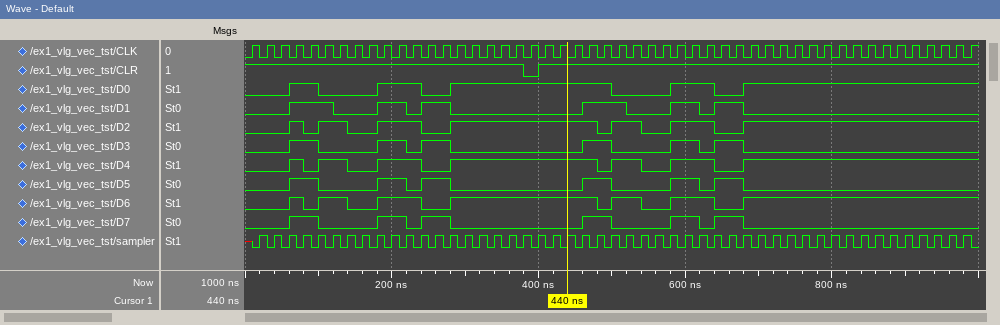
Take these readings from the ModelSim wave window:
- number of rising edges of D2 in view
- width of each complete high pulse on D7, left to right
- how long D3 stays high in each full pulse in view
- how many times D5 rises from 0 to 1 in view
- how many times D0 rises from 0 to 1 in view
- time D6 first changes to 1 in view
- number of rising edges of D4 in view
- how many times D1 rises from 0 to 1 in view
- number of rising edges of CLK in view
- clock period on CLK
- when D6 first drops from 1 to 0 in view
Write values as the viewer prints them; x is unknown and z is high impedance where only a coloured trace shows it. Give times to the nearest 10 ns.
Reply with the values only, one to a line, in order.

7
40 ns, 40 ns, 40 ns, 40 ns, 40 ns, 40 ns
40 ns, 40 ns, 40 ns, 40 ns, 40 ns, 40 ns
6
5
60 ns
7
6
50
20 ns
80 ns
